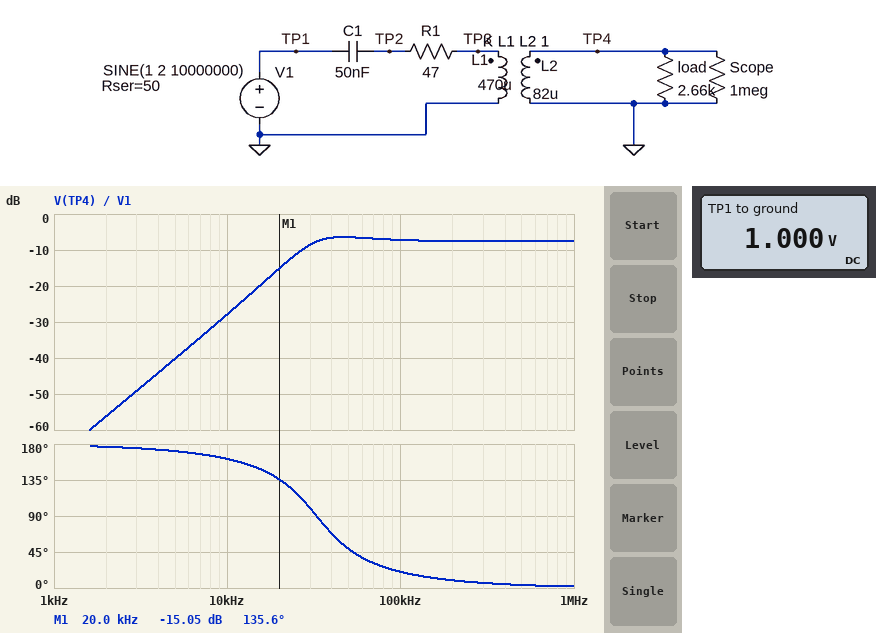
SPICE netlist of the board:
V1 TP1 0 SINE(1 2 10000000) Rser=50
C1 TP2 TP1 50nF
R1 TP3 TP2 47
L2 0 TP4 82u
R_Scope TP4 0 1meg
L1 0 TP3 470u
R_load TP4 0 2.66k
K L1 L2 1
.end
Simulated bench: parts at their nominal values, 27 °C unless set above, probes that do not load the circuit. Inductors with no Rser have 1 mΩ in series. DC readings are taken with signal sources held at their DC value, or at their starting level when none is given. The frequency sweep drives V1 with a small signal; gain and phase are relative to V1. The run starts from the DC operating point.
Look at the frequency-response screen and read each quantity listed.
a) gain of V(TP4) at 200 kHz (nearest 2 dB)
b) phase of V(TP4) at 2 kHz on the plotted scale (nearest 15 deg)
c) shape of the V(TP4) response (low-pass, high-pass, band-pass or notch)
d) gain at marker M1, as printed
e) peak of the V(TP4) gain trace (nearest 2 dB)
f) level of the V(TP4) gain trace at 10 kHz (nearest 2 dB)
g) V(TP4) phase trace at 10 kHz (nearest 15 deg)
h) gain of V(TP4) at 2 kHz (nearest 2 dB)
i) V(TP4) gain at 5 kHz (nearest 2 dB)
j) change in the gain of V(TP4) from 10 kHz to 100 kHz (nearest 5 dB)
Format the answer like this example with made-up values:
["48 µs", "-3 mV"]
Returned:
["-8 dB", "180 deg", "high-pass", "-15.05 dB", "-6 dB", "-28 dB", "165 deg", "-56 dB", "-40 dB", "20 dB"]
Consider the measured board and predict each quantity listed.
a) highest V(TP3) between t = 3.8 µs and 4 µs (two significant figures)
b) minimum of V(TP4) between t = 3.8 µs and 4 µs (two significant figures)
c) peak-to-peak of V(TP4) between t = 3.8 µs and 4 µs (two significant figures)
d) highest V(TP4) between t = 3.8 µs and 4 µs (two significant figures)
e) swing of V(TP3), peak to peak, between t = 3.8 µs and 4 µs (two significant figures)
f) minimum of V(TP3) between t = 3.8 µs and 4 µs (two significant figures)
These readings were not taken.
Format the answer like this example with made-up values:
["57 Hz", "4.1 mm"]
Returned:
["2.0 V", "-830 mV", "1.7 V", "830 mV", "4.0 V", "-2.0 V"]
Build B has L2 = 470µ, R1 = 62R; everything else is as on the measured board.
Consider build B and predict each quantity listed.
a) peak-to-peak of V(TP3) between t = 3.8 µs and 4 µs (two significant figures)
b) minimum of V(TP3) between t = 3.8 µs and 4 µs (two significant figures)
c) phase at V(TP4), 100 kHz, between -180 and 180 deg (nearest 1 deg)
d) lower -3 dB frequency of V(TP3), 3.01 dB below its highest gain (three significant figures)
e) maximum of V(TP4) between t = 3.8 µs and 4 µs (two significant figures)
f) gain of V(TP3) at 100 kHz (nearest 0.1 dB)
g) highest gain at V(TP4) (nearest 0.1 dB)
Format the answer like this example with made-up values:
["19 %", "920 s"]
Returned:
["3.8 V", "-1.9 V", "23 deg", "28.6 kHz", "1.9 V", "-0.1 dB", "0.1 dB"]
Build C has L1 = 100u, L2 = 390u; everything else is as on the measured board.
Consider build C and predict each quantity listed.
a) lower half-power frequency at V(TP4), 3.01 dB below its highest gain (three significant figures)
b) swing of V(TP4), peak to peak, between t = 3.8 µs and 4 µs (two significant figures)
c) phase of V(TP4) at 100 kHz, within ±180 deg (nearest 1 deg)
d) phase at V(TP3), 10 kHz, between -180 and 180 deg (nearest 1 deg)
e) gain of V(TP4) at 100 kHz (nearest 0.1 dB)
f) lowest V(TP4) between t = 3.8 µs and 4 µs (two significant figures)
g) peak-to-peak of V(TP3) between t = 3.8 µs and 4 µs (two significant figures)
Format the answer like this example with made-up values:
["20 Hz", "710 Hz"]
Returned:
["110 kHz", "6.9 V", "68 deg", "162 deg", "1.2 dB", "-3.5 V", "3.5 V"]
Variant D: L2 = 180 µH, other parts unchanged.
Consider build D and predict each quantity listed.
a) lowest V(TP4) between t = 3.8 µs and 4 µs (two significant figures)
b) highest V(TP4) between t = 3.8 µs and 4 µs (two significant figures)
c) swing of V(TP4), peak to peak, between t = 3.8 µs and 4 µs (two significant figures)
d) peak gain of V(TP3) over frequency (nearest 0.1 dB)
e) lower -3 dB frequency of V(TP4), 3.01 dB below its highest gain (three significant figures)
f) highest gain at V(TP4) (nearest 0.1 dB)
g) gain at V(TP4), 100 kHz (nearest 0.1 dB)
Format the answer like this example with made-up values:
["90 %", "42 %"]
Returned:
["-1.2 V", "1.2 V", "2.4 V", "1.1 dB", "27.9 kHz", "-3.1 dB", "-3.9 dB"]
